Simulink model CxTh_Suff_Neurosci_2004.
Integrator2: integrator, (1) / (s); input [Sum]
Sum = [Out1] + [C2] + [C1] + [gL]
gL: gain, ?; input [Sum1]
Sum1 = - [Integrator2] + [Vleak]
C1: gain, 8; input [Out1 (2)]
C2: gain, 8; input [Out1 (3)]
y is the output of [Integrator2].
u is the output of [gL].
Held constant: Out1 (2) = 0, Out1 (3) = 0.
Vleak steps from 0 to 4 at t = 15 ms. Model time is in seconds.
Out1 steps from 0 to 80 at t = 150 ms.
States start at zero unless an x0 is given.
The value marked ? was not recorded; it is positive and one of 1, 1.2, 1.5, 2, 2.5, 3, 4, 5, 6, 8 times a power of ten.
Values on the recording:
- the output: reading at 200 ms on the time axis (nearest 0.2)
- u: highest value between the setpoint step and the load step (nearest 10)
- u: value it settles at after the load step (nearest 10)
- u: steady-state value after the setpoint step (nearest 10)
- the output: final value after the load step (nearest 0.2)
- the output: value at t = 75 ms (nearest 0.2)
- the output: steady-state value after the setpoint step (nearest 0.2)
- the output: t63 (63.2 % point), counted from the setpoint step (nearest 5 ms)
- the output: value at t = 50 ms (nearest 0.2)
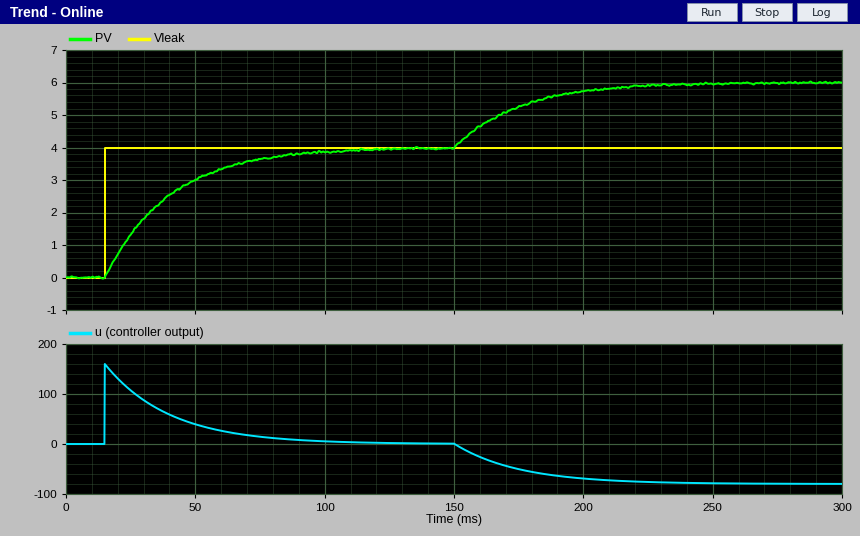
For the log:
5.8
160
-80
0
6.0
3.6
4.0
25 ms
3.0
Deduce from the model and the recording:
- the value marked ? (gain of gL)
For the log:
40
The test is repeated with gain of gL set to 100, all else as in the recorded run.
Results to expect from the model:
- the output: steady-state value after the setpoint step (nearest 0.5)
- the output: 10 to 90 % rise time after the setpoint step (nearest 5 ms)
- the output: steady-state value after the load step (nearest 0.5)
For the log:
4.0
20 ms
5.0
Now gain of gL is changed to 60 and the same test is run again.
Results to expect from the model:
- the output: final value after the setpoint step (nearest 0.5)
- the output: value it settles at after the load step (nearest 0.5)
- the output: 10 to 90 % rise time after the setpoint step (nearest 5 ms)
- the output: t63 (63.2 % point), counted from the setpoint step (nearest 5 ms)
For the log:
4.0
5.5
35 ms
15 ms
